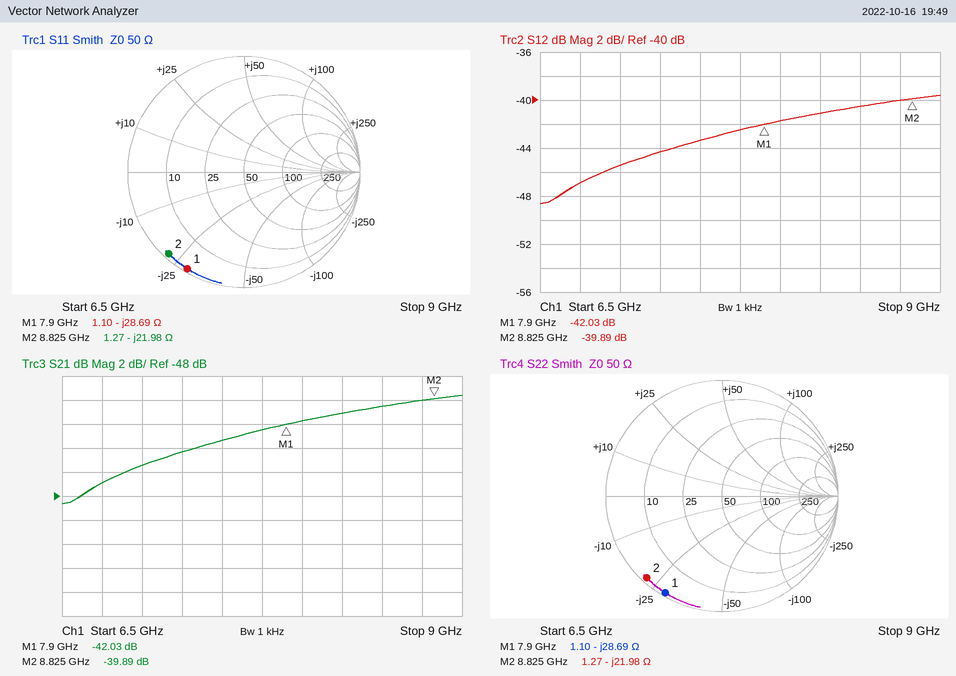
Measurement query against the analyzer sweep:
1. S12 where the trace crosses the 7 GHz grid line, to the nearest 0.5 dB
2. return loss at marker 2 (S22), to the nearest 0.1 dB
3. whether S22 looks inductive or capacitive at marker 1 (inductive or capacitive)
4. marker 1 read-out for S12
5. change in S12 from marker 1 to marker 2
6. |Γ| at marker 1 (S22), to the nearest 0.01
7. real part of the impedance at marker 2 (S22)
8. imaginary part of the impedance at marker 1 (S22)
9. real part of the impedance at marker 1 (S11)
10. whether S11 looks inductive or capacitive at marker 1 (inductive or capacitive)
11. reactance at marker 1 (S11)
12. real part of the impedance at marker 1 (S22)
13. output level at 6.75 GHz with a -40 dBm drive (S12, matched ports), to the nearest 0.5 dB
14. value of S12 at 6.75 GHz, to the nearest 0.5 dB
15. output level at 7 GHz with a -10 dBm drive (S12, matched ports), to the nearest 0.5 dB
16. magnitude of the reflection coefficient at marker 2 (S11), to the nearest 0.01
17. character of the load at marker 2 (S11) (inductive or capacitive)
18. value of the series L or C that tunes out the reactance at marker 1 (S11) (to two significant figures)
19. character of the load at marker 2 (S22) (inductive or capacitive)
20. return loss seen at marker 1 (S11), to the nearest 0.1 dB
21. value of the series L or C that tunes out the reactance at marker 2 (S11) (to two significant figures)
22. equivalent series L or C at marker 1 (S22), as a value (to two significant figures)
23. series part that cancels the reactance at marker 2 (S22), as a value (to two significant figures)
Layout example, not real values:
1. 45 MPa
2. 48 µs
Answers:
1. -45.5 dB
2. 0.4 dB
3. capacitive
4. -42.03 dB
5. 2.14 dB
6. 0.97
7. 1.27 Ω
8. -28.69 Ω
9. 1.10 Ω
10. capacitive
11. -28.69 Ω
12. 1.10 Ω
13. -87.0 dBm
14. -47.0 dB
15. -55.5 dBm
16. 0.96
17. capacitive
18. 580 pH
19. capacitive
20. 0.3 dB
21. 400 pH
22. 700 fF
23. 400 pH
